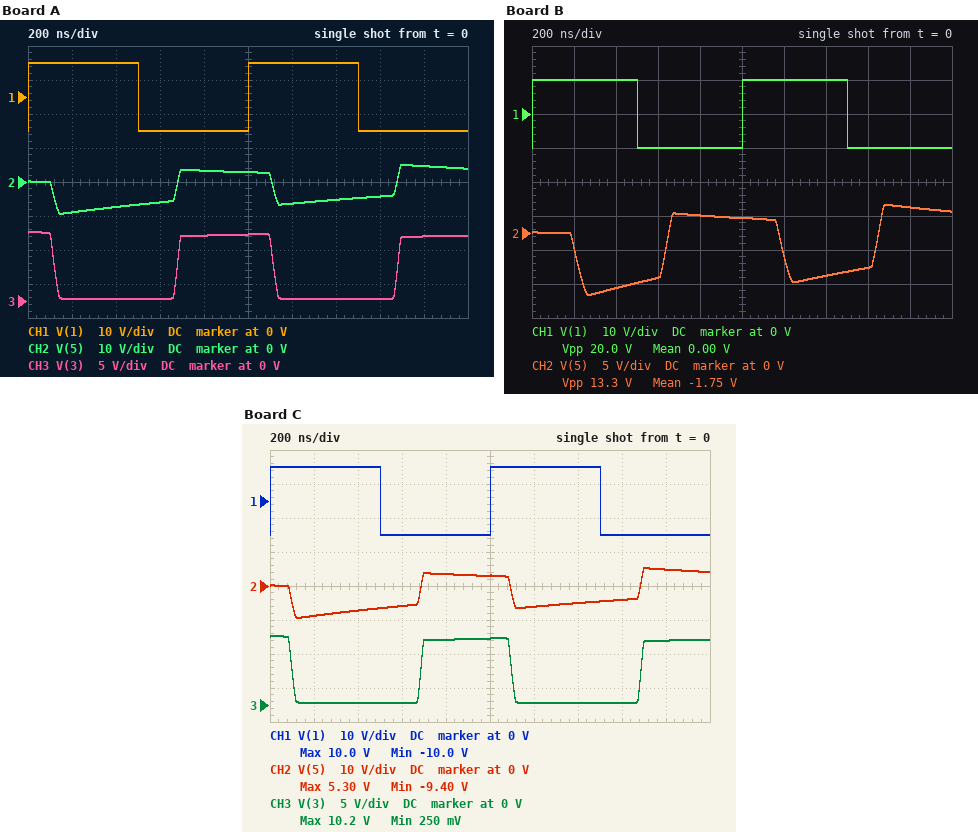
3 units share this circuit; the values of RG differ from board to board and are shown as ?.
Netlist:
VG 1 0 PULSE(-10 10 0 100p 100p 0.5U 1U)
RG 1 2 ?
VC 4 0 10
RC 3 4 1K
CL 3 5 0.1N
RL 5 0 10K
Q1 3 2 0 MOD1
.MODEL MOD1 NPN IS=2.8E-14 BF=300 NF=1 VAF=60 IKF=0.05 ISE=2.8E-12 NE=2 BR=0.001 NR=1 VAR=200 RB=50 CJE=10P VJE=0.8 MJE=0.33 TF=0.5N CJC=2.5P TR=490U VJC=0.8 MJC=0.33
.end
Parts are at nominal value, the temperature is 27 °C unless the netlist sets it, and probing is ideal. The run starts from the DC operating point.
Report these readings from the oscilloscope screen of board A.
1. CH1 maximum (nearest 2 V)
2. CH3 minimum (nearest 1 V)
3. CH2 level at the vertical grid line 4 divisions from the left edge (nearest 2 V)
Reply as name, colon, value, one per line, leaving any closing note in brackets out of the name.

CH1 maximum: 10 V
CH3 minimum: 0 V
CH2 level at the vertical grid line 4 divisions from the left edge: 4 V
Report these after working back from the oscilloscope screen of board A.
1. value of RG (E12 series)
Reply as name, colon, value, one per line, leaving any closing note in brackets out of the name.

value of RG: 18 kΩ
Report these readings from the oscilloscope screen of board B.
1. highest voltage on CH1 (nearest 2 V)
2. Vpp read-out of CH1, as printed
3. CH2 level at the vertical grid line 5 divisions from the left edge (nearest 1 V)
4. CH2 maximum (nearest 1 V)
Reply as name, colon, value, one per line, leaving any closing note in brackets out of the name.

highest voltage on CH1: 10 V
Vpp read-out of CH1, as printed: 20.0 V
CH2 level at the vertical grid line 5 divisions from the left edge: 2 V
CH2 maximum: 4 V
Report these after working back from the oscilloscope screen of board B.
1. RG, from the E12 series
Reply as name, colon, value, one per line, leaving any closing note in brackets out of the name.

RG, from the E12 series: 33 kΩ
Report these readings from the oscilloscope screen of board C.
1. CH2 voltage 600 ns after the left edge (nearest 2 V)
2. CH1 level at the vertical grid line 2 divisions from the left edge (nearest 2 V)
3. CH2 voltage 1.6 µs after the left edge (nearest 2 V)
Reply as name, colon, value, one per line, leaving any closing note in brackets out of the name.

CH2 voltage 600 ns after the left edge: -6 V
CH1 level at the vertical grid line 2 divisions from the left edge: 10 V
CH2 voltage 1.6 µs after the left edge: -4 V
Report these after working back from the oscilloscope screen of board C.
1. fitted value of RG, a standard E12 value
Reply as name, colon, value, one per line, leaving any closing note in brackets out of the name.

fitted value of RG, a standard E12 value: 15 kΩ
